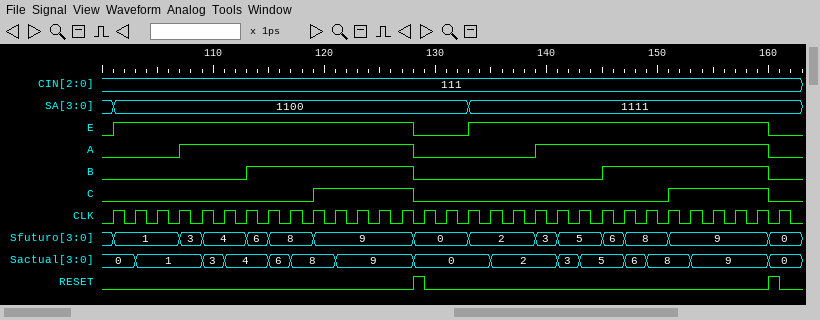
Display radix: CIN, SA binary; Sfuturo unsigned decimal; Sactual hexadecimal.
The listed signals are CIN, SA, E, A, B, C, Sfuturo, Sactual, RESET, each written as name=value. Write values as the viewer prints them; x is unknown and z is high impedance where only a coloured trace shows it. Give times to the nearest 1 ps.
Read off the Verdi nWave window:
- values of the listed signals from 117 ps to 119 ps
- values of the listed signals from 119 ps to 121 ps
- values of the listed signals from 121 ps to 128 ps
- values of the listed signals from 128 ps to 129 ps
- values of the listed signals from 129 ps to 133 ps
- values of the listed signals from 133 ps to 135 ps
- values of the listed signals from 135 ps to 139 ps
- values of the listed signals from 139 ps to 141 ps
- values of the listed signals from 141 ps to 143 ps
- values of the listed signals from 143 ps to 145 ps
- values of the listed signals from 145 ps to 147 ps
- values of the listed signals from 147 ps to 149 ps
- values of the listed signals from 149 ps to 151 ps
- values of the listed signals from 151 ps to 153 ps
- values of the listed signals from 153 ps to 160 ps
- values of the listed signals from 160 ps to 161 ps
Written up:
CIN=111, SA=1100, E=1, A=1, B=1, C=0, Sfuturo=8, Sactual=8, RESET=0
CIN=111, SA=1100, E=1, A=1, B=1, C=1, Sfuturo=9, Sactual=8, RESET=0
CIN=111, SA=1100, E=1, A=1, B=1, C=1, Sfuturo=9, Sactual=9, RESET=0
CIN=111, SA=1100, E=0, A=0, B=0, C=0, Sfuturo=0, Sactual=0, RESET=1
CIN=111, SA=1100, E=0, A=0, B=0, C=0, Sfuturo=0, Sactual=0, RESET=0
CIN=111, SA=1111, E=1, A=0, B=0, C=0, Sfuturo=2, Sactual=0, RESET=0
CIN=111, SA=1111, E=1, A=0, B=0, C=0, Sfuturo=2, Sactual=2, RESET=0
CIN=111, SA=1111, E=1, A=1, B=0, C=0, Sfuturo=3, Sactual=2, RESET=0
CIN=111, SA=1111, E=1, A=1, B=0, C=0, Sfuturo=5, Sactual=3, RESET=0
CIN=111, SA=1111, E=1, A=1, B=0, C=0, Sfuturo=5, Sactual=5, RESET=0
CIN=111, SA=1111, E=1, A=1, B=1, C=0, Sfuturo=6, Sactual=5, RESET=0
CIN=111, SA=1111, E=1, A=1, B=1, C=0, Sfuturo=8, Sactual=6, RESET=0
CIN=111, SA=1111, E=1, A=1, B=1, C=0, Sfuturo=8, Sactual=8, RESET=0
CIN=111, SA=1111, E=1, A=1, B=1, C=1, Sfuturo=9, Sactual=8, RESET=0
CIN=111, SA=1111, E=1, A=1, B=1, C=1, Sfuturo=9, Sactual=9, RESET=0
CIN=111, SA=1111, E=0, A=0, B=0, C=0, Sfuturo=0, Sactual=0, RESET=1
